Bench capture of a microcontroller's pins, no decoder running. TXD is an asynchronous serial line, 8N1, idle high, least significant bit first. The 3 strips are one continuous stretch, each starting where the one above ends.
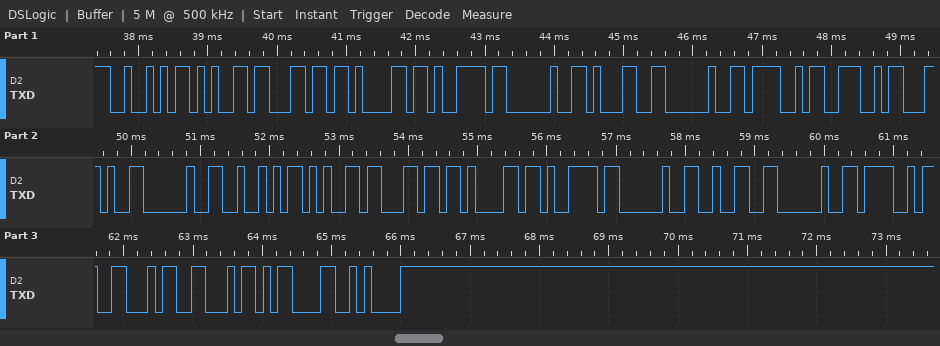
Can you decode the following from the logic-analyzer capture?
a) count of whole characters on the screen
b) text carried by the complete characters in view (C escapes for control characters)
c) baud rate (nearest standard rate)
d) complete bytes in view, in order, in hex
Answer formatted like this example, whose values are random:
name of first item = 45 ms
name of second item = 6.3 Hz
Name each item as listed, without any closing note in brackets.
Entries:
count of whole characters on the screen = 25
text carried by the complete characters in view = "Relay 1 ON, Relay 2 OFF\r\n"
baud rate = 9600 baud
complete bytes in view, in order, in hex = 52 65 6C 61 79 20 31 20 4F 4E 2C 20 52 65 6C 61 79 20 32 20 4F 46 46 0D 0A
